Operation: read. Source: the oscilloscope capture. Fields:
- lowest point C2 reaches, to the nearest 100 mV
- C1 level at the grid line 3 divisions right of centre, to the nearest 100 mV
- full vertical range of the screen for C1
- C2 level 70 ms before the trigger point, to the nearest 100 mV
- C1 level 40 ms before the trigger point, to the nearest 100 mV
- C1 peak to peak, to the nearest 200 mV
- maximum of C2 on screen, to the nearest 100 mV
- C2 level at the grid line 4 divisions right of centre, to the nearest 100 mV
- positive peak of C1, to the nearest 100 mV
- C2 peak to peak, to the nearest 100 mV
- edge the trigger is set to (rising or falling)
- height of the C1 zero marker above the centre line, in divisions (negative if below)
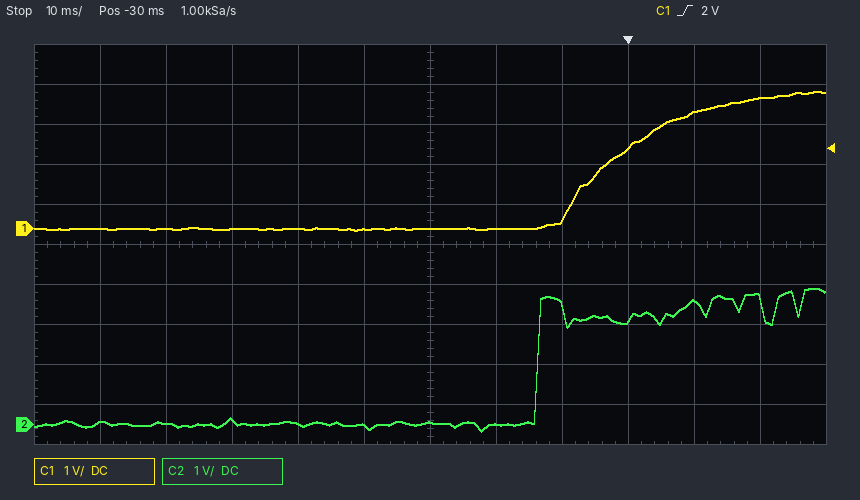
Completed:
-200 mV
2.0 V
10 V
0.0 V
0.0 V
3.4 V
3.4 V
3.1 V
3.4 V
3.6 V
rising
+0.4 div
